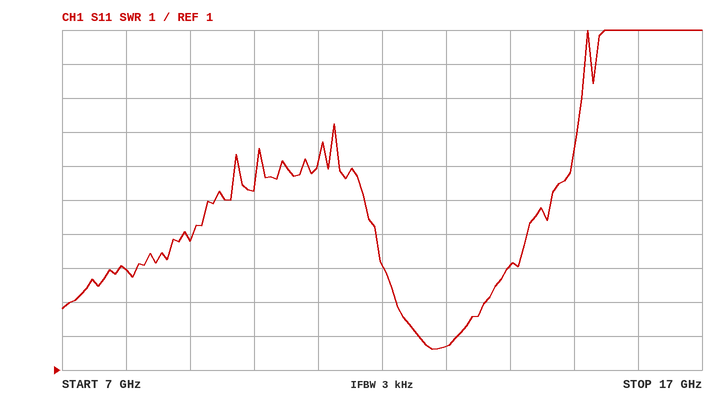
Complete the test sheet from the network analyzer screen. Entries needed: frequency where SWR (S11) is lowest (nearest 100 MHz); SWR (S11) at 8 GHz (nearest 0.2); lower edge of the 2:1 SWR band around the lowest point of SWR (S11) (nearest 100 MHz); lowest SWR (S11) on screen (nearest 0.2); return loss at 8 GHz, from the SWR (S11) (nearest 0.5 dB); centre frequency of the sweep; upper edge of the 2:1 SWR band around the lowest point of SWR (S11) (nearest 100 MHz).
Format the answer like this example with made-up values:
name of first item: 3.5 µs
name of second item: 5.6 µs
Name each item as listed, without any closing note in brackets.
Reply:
frequency where SWR (S11) is lowest: 12.8 GHz
SWR (S11) at 8 GHz: 4.0
lower edge of the 2:1 SWR band around the lowest point of SWR (S11): 12.6 GHz
lowest SWR (S11) on screen: 1.6
return loss at 8 GHz, from the SWR (S11): 4.5 dB
centre frequency of the sweep: 12 GHz
upper edge of the 2:1 SWR band around the lowest point of SWR (S11): 13.2 GHz
